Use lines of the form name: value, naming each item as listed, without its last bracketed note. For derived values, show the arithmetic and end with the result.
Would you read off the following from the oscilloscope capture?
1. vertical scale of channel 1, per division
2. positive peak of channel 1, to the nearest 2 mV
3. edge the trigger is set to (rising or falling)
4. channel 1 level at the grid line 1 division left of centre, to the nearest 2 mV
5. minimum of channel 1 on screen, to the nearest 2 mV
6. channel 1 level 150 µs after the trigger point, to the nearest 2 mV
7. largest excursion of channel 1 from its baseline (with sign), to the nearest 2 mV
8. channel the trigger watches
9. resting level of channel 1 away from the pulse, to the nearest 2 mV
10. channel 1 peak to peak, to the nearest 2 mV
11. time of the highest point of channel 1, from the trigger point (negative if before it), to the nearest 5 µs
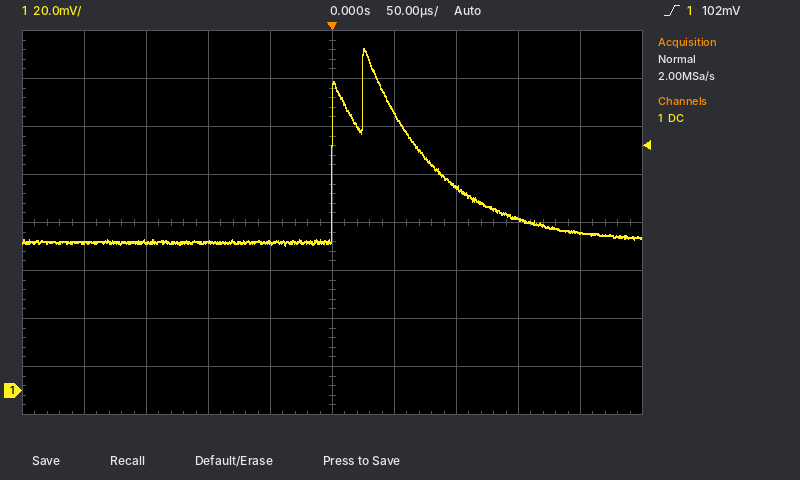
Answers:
vertical scale of channel 1, per division: 20 mV
positive peak of channel 1, to the nearest 2 mV: 142 mV
edge the trigger is set to: rising
channel 1 level at the grid line 1 division left of centre, to the nearest 2 mV: 62 mV
minimum of channel 1 on screen, to the nearest 2 mV: 60 mV
channel 1 level 150 µs after the trigger point, to the nearest 2 mV: 72 mV
largest excursion of channel 1 from its baseline (with sign), to the nearest 2 mV: 142 mV − (62 mV) = +80 mV
channel the trigger watches: channel 1
resting level of channel 1 away from the pulse, to the nearest 2 mV: 62 mV
channel 1 peak to peak, to the nearest 2 mV: 142 mV − (60 mV) = 82 mV
time of the highest point of channel 1, from the trigger point (negative if before it), to the nearest 5 µs: +25 µs
